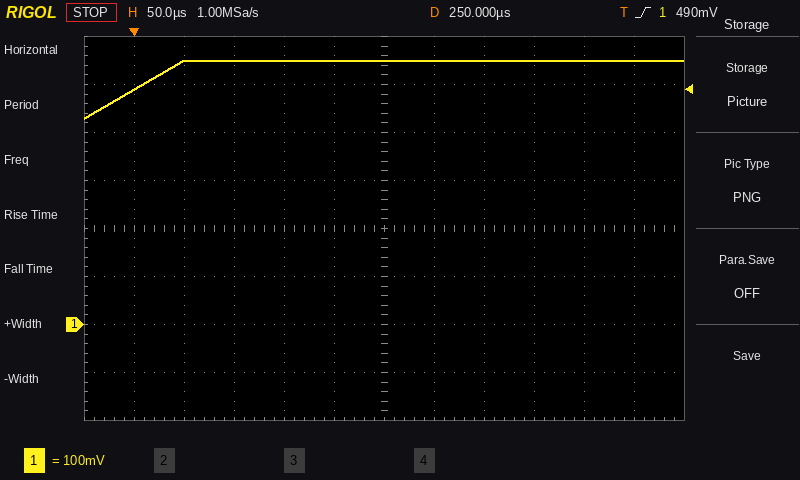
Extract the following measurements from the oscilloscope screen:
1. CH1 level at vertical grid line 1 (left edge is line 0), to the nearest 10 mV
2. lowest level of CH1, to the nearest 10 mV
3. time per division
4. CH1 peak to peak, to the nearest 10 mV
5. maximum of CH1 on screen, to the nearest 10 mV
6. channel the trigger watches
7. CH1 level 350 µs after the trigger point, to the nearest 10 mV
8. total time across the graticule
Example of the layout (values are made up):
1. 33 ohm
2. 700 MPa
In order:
1. 490 mV
2. 430 mV
3. 50 µs
4. 120 mV
5. 550 mV
6. CH1
7. 550 mV
8. 600 µs
